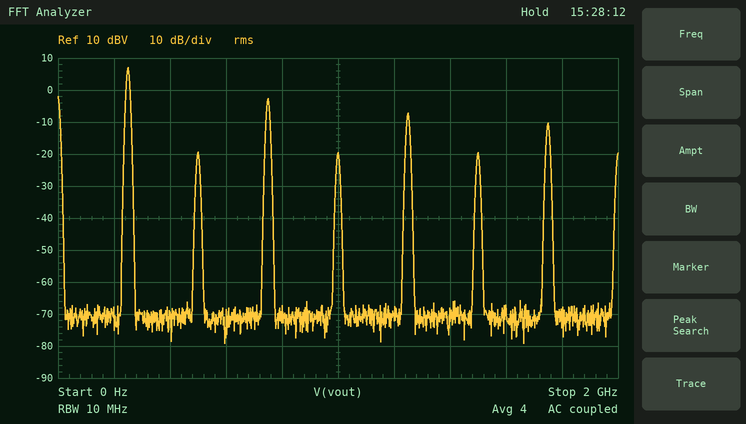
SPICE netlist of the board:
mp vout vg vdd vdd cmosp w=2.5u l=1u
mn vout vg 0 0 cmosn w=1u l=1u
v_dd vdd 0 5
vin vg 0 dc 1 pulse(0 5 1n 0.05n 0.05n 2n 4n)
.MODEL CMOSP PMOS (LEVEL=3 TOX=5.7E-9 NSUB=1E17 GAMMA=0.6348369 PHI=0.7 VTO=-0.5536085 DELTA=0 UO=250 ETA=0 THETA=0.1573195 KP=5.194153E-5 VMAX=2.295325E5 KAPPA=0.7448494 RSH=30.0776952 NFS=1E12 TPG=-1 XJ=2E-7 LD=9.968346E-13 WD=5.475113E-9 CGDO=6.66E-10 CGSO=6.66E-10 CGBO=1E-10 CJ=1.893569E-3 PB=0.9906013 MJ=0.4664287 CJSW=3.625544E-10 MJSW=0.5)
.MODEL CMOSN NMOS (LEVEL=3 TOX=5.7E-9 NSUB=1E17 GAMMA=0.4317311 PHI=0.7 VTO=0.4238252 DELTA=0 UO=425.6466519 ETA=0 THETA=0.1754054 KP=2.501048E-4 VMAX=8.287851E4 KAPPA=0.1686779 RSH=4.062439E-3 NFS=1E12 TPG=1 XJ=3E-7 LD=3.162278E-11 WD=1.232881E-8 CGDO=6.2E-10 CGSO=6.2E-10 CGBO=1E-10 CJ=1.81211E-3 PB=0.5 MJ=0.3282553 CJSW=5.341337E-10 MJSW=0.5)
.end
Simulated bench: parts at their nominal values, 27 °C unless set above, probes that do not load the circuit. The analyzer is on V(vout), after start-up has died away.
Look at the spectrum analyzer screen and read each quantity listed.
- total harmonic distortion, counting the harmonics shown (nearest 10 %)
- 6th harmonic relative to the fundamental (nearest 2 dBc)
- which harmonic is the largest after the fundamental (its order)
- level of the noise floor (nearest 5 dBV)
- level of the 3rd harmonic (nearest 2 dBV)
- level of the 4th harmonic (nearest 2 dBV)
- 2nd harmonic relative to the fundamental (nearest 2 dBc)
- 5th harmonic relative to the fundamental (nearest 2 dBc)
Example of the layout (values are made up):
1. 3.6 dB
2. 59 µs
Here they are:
1. 40 %
2. -26 dBc
3. 3
4. -70 dBV
5. -2 dBV
6. -20 dBV
7. -26 dBc
8. -14 dBc
